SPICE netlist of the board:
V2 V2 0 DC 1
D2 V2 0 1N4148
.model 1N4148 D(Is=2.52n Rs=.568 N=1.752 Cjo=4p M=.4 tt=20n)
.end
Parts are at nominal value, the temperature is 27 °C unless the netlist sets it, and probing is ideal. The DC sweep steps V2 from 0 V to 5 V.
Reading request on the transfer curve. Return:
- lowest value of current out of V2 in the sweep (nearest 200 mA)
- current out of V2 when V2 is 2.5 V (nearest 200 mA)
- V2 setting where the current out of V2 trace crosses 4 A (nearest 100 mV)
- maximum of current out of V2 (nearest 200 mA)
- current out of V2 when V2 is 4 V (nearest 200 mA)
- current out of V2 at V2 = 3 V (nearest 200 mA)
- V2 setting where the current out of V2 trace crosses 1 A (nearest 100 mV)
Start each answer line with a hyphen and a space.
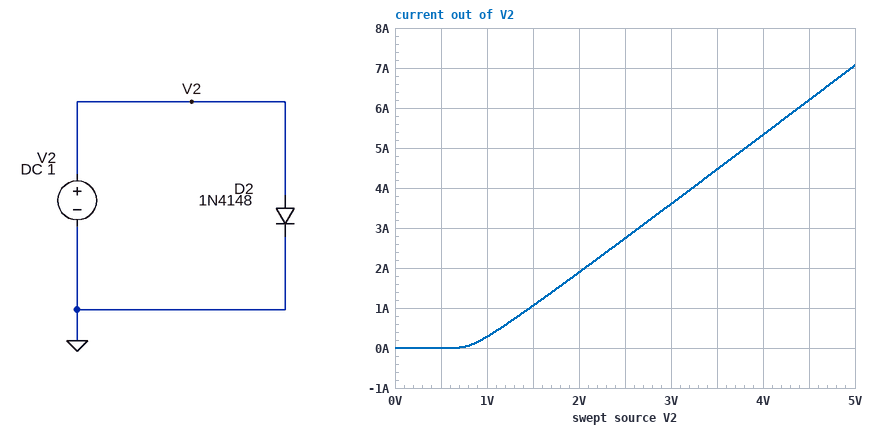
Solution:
- 0 A
- 2.8 A
- 3.2 V
- 7.0 A
- 5.4 A
- 3.6 A
- 1.5 V
